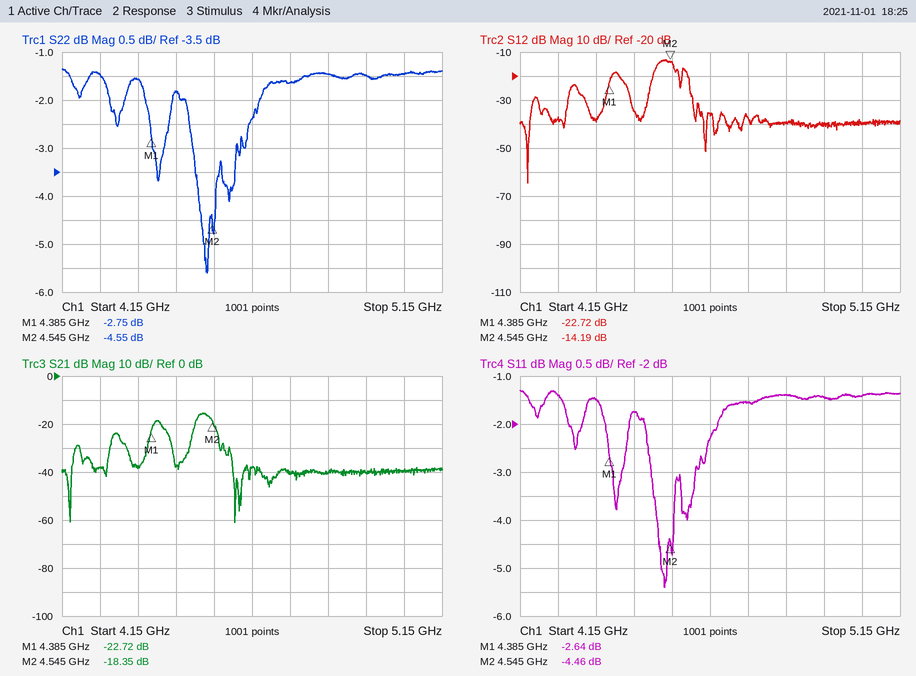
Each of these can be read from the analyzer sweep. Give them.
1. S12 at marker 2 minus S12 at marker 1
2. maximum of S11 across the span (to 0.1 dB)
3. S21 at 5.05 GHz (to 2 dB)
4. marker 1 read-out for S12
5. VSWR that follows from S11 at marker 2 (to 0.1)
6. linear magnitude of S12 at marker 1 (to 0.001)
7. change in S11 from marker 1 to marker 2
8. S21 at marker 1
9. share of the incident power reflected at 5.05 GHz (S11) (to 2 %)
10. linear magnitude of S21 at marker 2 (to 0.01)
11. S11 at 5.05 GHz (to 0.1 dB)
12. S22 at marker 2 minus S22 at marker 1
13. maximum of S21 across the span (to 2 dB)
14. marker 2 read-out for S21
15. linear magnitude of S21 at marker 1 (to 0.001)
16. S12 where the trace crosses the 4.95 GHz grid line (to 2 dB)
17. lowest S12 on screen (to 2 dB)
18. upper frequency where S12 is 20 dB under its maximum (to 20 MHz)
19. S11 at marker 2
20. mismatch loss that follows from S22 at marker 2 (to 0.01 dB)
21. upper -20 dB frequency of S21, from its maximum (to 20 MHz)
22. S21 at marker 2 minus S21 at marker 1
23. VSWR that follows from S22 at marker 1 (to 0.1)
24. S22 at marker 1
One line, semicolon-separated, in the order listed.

8.53 dB; -1.3 dB; -40 dB; -22.72 dB; 4.0; 0.073; -1.82 dB; -22.72 dB; 72 %; 0.12; -1.4 dB; -1.80 dB; -16 dB; -18.35 dB; 0.073; -40 dB; -64 dB; 4.60 GHz; -4.46 dB; 1.88 dB; 4.60 GHz; 4.37 dB; 6.4; -2.75 dB
